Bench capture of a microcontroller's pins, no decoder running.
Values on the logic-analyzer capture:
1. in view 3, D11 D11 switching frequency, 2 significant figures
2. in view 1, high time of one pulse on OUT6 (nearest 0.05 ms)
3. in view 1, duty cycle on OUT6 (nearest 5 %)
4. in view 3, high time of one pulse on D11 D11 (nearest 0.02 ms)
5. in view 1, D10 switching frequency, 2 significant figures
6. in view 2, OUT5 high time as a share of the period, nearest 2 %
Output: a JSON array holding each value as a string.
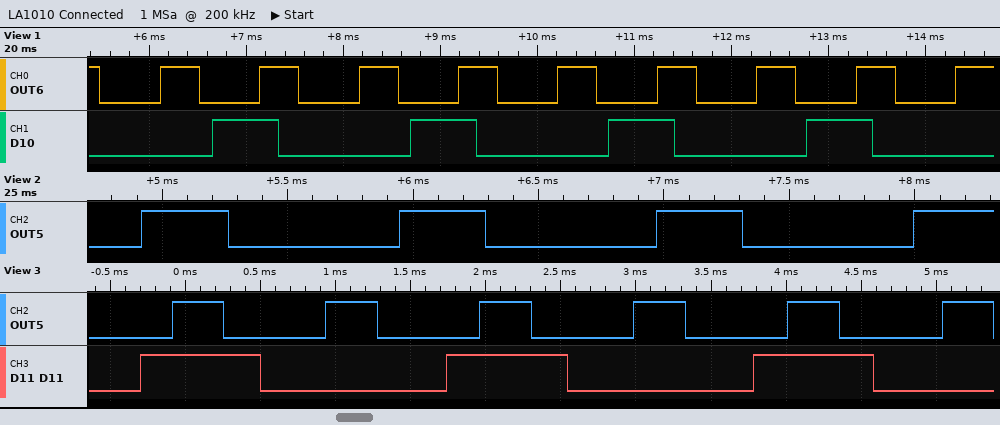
["490 Hz", "0.40 ms", "40 %", "0.80 ms", "490 Hz", "34 %"]
